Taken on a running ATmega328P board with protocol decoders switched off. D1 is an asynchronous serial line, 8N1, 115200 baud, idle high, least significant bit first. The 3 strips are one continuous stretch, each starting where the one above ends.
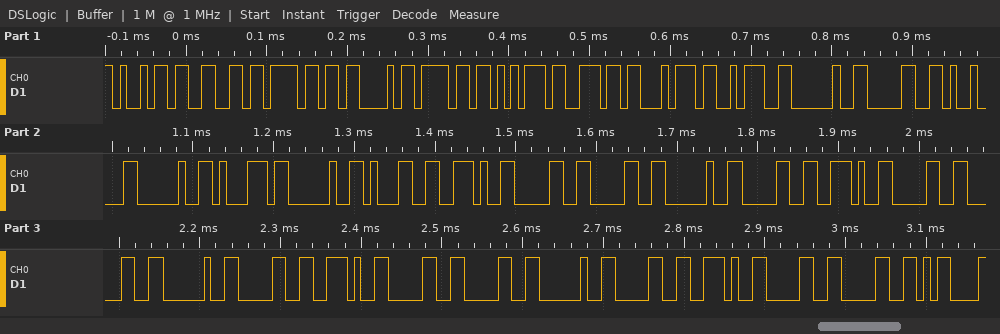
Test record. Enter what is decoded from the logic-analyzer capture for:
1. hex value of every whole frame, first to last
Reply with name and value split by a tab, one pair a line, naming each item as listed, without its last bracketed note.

hex value of every whole frame, first to last	69 66 6F 43 6F 75 6E 74 3A 20 30 09 20 71 20 31 2E 30 30 20 30 2E 30 30 20 30 2E 30 30 20 30 2E 30 30 0D
